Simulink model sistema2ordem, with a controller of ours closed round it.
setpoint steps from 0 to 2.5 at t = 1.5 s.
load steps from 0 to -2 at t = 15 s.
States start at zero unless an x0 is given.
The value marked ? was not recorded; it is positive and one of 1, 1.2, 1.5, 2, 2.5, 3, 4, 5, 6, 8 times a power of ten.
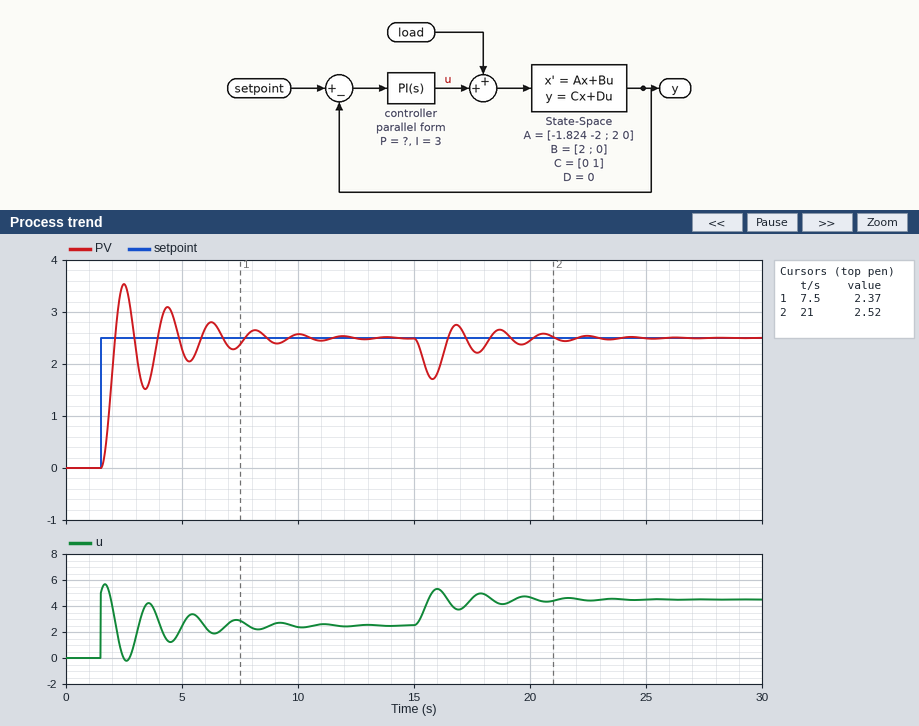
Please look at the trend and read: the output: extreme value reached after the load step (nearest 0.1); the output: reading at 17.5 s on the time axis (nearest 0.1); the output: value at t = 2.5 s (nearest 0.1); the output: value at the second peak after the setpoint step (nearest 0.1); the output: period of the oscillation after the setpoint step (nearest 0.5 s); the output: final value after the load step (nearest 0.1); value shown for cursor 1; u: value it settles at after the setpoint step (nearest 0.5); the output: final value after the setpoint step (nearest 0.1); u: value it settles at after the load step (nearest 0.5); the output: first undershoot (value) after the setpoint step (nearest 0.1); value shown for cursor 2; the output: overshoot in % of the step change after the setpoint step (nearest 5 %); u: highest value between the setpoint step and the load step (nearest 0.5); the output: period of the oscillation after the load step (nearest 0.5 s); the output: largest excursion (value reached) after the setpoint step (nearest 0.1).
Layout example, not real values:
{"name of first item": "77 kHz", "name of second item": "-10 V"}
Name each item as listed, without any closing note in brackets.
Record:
{"the output: extreme value reached after the load step": "1.7", "the output: reading at 17.5 s on the time axis": "2.3", "the output: value at t = 2.5 s": "3.5", "the output: value at the second peak after the setpoint step": "3.1", "the output: period of the oscillation after the setpoint step": "2.0 s", "the output: final value after the load step": "2.5", "value shown for cursor 1": "2.37", "u: value it settles at after the setpoint step": "2.5", "the output: final value after the setpoint step": "2.5", "u: value it settles at after the load step": "4.5", "the output: first undershoot (value) after the setpoint step": "1.5", "value shown for cursor 2": "2.52", "the output: overshoot in % of the step change after the setpoint step": "40 %", "u: highest value between the setpoint step and the load step": "5.5", "the output: period of the oscillation after the load step": "2.0 s", "the output: largest excursion (value reached) after the setpoint step": "3.5"}
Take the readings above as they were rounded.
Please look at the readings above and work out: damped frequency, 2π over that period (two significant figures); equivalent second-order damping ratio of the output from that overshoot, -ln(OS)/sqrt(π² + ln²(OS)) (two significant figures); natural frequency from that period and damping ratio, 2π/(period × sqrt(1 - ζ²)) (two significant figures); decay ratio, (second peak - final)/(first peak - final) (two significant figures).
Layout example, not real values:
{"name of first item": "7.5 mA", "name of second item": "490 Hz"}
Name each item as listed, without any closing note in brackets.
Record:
{"damped frequency, 2π over that period": "3.1 rad/s", "equivalent second-order damping ratio of the output from that overshoot, -ln(OS)/sqrt(π² + ln²(OS))": "0.28", "natural frequency from that period and damping ratio, 2π/(period × sqrt(1 - ζ²))": "3.3 rad/s", "decay ratio, (second peak - final)/(first peak - final)": "0.60"}
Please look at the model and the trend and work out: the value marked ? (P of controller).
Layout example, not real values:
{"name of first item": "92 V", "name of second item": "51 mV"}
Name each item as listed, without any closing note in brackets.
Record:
{"the value marked ?": "2"}
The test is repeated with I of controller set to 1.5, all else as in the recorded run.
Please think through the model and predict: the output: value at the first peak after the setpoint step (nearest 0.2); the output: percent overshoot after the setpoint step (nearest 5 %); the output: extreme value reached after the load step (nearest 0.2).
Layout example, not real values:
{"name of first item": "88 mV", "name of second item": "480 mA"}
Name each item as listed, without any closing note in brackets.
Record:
{"the output: value at the first peak after the setpoint step": "3.0", "the output: percent overshoot after the setpoint step": "20 %", "the output: extreme value reached after the load step": "1.6"}
